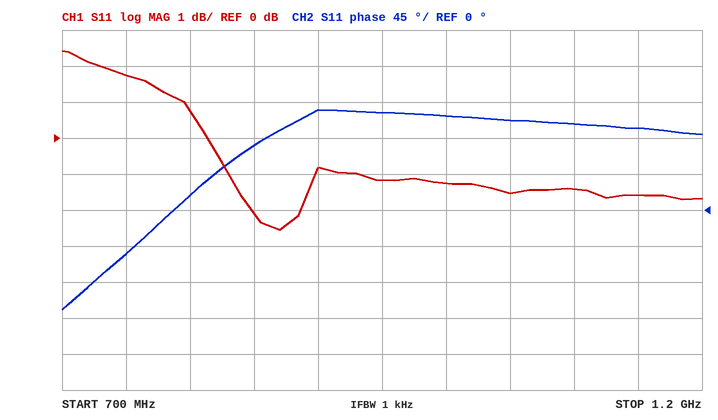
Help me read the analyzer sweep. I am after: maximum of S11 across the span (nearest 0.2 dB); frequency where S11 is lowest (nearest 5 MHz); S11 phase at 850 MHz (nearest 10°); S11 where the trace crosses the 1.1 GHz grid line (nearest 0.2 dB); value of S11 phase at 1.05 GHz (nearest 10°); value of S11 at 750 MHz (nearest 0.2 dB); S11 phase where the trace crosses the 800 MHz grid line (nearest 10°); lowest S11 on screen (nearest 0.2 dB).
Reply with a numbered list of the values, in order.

1. 2.4 dB
2. 870 MHz
3. 80°
4. -1.4 dB
5. 110°
6. 1.8 dB
7. 20°
8. -2.6 dB
